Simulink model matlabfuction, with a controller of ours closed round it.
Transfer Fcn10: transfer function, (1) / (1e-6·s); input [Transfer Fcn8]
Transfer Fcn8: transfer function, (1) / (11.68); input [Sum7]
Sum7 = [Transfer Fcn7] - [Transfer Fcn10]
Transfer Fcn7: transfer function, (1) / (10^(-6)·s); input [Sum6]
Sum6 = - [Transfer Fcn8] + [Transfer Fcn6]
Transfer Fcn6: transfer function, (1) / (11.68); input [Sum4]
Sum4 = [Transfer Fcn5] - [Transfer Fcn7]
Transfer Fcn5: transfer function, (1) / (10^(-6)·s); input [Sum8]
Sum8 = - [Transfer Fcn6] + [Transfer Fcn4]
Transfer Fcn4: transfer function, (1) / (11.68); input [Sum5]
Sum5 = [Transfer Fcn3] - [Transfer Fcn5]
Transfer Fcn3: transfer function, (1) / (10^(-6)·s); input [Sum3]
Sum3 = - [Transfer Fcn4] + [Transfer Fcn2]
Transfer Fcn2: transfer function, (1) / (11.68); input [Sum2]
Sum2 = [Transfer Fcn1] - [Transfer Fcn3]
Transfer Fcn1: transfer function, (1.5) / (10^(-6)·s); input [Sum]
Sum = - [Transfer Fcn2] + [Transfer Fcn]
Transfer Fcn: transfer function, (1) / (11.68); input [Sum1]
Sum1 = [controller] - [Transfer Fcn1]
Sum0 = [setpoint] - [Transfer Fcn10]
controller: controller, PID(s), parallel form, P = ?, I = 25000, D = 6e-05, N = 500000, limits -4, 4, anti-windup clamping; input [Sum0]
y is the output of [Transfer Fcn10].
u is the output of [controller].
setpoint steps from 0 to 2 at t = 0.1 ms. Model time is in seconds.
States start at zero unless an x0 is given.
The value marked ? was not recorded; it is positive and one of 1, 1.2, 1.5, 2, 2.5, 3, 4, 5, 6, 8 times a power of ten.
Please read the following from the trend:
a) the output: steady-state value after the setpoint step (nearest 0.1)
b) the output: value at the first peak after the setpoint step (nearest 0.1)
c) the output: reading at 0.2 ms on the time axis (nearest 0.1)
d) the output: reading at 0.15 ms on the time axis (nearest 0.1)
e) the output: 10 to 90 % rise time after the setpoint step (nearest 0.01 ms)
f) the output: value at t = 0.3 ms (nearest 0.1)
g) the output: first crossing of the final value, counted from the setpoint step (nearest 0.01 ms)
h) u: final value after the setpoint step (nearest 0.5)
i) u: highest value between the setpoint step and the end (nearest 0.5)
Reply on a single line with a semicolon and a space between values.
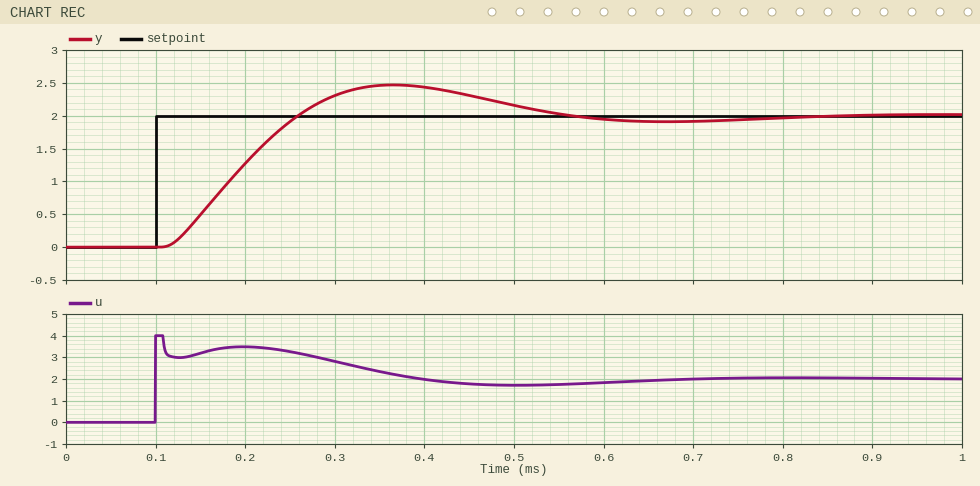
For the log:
2.0; 2.5; 1.3; 0.5; 0.11 ms; 2.3; 0.16 ms; 2.0; 4.0
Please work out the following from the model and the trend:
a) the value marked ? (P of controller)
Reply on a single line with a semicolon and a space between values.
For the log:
1.5
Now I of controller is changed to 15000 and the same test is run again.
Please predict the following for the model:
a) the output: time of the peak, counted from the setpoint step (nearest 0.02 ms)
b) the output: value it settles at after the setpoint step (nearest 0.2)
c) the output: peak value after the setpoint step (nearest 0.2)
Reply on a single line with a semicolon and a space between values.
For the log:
0.34 ms; 2.0; 2.2
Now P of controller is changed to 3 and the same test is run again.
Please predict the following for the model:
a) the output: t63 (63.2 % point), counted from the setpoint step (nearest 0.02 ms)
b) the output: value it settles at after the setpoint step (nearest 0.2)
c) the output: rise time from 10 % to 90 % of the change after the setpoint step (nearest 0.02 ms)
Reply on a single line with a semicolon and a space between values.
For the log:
0.08 ms; 2.0; 0.12 ms
